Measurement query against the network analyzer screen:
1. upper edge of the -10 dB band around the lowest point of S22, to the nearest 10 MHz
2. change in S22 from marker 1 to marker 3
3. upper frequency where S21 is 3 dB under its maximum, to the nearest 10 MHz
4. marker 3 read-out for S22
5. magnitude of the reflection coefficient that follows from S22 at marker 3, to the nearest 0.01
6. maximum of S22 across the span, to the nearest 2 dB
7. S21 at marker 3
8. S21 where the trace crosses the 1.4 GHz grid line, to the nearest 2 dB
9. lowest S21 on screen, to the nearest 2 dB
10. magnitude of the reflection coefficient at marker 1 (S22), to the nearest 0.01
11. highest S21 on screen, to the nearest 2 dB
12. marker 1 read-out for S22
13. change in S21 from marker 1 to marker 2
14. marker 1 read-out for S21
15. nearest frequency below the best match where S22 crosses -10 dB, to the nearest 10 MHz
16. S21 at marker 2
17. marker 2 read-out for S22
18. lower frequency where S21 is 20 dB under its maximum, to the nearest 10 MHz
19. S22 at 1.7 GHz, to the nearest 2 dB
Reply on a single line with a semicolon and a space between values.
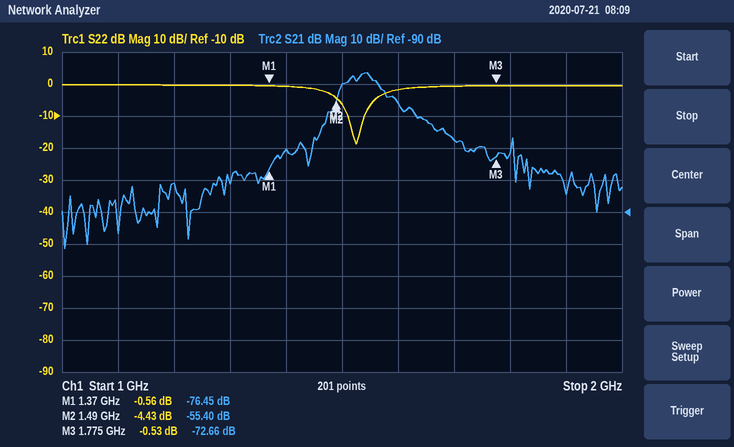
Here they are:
1.54 GHz; 0.03 dB; 1.56 GHz; -0.53 dB; 0.94; 0 dB; -72.66 dB; -70 dB; -102 dB; 0.94; -46 dB; -0.56 dB; 21.05 dB; -76.45 dB; 1.51 GHz; -55.40 dB; -4.43 dB; 1.46 GHz; 0 dB
